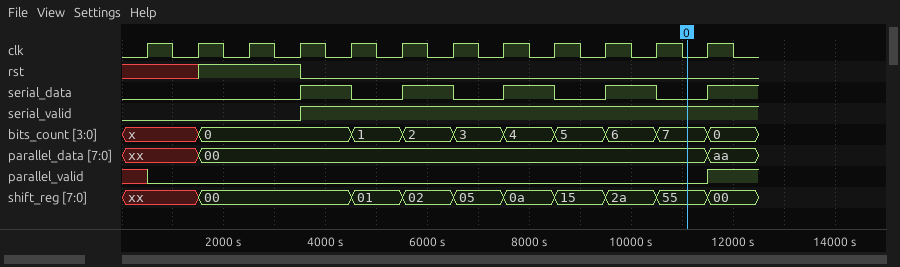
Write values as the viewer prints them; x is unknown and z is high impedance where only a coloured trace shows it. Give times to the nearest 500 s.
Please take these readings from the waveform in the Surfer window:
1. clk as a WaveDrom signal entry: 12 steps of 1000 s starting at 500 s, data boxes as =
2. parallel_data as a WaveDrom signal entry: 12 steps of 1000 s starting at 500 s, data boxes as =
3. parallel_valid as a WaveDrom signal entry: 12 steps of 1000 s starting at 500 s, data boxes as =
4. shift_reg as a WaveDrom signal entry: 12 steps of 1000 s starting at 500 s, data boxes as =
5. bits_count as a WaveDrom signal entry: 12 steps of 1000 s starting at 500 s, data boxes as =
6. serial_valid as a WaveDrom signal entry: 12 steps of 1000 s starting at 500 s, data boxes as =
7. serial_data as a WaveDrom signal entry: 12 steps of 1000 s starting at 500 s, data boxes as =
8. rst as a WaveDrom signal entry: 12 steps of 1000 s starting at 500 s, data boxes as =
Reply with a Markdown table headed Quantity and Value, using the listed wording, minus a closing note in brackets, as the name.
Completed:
| Quantity | Value |
|---|---|
| clk as a WaveDrom signal entry: 12 steps of 1000 s starting at 500 s, data boxes as = | {name: 'clk', wave: 'p...........'} |
| parallel_data as a WaveDrom signal entry: 12 steps of 1000 s starting at 500 s, data boxes as = | {name: 'parallel_data', wave: 'x=.........=', data: '00 aa'} |
| parallel_valid as a WaveDrom signal entry: 12 steps of 1000 s starting at 500 s, data boxes as = | {name: 'parallel_valid', wave: '0..........1'} |
| shift_reg as a WaveDrom signal entry: 12 steps of 1000 s starting at 500 s, data boxes as = | {name: 'shift_reg', wave: 'x=..========', data: '00 01 02 05 0a 15 2a 55 00'} |
| bits_count as a WaveDrom signal entry: 12 steps of 1000 s starting at 500 s, data boxes as = | {name: 'bits_count', wave: 'x=..========', data: '0 1 2 3 4 5 6 7 0'} |
| serial_valid as a WaveDrom signal entry: 12 steps of 1000 s starting at 500 s, data boxes as = | {name: 'serial_valid', wave: '0..1........'} |
| serial_data as a WaveDrom signal entry: 12 steps of 1000 s starting at 500 s, data boxes as = | {name: 'serial_data', wave: '0..101010101'} |
| rst as a WaveDrom signal entry: 12 steps of 1000 s starting at 500 s, data boxes as = | {name: 'rst', wave: 'x1.0........'} |
